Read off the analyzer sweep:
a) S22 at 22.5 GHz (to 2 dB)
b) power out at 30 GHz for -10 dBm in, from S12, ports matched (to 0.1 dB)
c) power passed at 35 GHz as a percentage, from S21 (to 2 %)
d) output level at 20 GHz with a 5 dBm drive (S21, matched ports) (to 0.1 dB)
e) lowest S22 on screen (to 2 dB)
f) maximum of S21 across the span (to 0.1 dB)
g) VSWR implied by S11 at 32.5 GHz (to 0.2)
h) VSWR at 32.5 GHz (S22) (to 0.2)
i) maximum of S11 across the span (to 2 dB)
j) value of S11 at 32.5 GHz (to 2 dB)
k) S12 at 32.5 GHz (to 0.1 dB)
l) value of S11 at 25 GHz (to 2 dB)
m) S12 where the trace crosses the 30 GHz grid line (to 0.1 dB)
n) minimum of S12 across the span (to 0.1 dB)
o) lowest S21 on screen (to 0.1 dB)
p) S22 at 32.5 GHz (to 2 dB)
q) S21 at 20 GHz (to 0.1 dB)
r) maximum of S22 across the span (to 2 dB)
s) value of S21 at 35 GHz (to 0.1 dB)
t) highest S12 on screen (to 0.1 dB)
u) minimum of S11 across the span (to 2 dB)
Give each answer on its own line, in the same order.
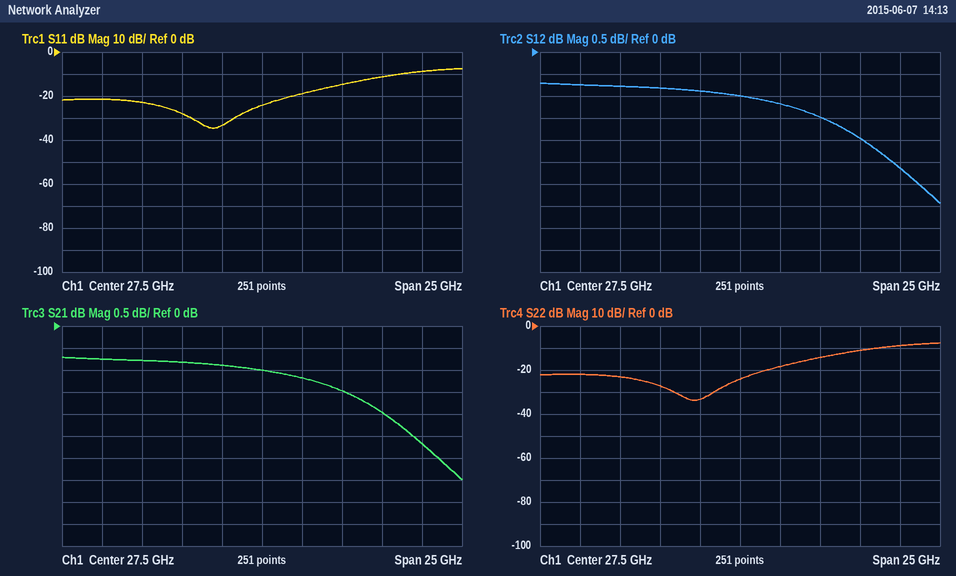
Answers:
-28 dB
-11.2 dBm
64 %
4.2 dBm
-34 dB
-0.7 dB
1.4
1.4
-8 dB
-14 dB
-1.5 dB
-34 dB
-1.2 dB
-3.4 dB
-3.5 dB
-14 dB
-0.8 dB
-8 dB
-2.0 dB
-0.7 dB
-34 dB
